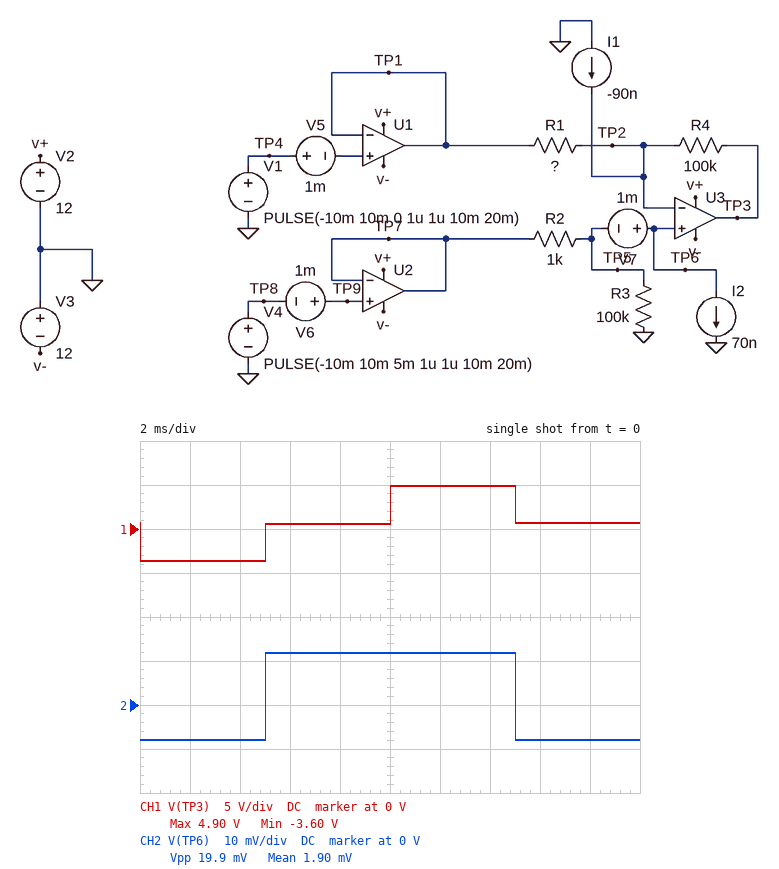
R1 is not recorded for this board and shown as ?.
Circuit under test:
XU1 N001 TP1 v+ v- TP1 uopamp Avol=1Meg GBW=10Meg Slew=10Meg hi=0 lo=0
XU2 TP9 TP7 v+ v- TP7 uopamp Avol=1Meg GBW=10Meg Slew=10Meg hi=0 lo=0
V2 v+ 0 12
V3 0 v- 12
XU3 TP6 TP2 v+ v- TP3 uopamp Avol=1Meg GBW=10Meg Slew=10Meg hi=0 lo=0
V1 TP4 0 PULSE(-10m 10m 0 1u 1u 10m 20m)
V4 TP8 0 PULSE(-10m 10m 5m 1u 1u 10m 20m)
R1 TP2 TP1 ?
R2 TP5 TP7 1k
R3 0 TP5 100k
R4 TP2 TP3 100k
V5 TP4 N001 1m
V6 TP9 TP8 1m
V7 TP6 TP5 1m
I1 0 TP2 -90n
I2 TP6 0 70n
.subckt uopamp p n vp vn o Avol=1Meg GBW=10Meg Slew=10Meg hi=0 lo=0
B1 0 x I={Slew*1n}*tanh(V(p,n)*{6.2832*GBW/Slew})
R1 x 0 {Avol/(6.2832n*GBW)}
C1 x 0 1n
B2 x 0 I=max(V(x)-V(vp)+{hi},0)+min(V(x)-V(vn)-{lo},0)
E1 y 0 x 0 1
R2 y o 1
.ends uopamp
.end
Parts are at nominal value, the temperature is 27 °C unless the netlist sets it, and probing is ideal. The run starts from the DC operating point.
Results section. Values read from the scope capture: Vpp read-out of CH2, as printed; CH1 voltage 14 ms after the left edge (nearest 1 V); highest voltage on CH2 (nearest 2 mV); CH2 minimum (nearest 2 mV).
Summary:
19.9 mV
5 V
12 mV
-8 mV
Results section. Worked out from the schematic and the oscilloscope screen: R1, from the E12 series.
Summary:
470 Ω
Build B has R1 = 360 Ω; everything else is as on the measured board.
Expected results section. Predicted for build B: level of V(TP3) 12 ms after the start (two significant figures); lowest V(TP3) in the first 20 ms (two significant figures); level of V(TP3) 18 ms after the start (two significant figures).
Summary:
6.4 V
-4.7 V
840 mV
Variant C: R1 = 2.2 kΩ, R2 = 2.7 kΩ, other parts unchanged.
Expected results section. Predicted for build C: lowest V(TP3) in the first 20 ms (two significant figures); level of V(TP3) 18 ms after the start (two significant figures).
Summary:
-770 mV
140 mV
